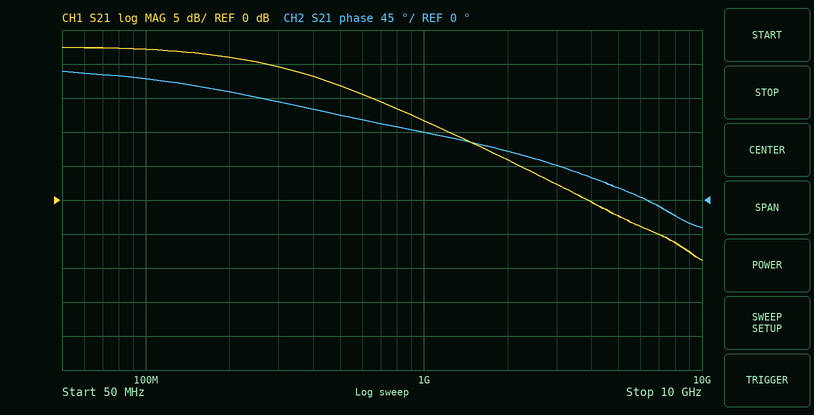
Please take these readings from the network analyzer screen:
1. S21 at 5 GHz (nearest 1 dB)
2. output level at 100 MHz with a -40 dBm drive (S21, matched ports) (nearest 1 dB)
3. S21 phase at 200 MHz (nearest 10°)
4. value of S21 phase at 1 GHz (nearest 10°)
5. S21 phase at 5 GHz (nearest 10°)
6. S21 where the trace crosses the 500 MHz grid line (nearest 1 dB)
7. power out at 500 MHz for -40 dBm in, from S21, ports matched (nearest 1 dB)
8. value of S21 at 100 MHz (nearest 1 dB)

-2 dB
-18 dBm
140°
90°
20°
17 dB
-23 dBm
22 dB
